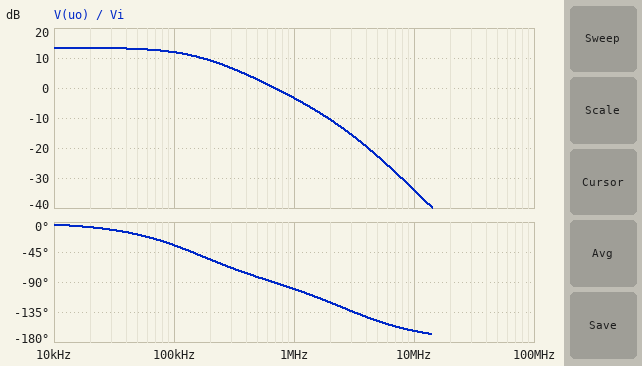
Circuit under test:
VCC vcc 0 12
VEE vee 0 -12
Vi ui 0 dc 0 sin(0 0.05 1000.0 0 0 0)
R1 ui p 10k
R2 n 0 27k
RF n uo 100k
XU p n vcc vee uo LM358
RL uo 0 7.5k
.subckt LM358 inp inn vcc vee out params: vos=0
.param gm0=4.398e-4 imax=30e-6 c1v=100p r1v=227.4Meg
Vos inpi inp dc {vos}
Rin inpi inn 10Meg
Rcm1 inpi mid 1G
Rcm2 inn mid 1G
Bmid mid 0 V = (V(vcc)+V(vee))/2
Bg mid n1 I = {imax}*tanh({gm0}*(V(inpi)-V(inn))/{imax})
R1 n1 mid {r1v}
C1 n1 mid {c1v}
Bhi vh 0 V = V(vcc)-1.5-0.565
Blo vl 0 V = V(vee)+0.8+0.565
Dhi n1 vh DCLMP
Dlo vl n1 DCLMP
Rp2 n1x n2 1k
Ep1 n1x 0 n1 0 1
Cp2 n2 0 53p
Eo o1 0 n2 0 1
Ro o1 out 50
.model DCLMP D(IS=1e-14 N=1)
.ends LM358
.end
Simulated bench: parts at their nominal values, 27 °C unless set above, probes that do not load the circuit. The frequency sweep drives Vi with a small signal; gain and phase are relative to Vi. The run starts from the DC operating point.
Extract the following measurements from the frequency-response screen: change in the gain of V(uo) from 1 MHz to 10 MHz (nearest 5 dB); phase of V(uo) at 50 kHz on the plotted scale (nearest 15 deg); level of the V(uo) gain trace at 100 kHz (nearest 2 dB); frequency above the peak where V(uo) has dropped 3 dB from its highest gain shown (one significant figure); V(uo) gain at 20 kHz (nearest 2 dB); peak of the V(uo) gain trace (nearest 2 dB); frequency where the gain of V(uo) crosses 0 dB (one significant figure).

-30 dB
-15 deg
12 dB
200 kHz
14 dB
14 dB
700 kHz
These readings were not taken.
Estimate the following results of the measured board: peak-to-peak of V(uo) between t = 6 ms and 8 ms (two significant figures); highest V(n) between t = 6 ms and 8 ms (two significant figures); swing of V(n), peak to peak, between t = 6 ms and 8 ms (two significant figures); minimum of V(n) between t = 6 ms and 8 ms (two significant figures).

470 mV
50 mV
100 mV
-50 mV
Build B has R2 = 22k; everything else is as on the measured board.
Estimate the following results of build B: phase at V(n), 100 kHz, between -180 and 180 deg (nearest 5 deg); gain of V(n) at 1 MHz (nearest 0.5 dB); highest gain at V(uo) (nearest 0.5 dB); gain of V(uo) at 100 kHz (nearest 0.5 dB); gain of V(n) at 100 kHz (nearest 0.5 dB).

-40 deg
-18.5 dB
15.0 dB
13.0 dB
-2.0 dB
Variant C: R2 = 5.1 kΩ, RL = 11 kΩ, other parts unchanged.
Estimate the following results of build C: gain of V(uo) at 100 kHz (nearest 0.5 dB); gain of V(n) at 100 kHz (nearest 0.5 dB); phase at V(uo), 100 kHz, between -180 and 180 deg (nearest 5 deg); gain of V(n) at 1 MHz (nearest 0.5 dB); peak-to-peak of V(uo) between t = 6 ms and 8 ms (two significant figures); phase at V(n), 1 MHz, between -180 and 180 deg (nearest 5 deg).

16.5 dB
-10.0 dB
-75 deg
-30.0 dB
2.1 V
-105 deg
